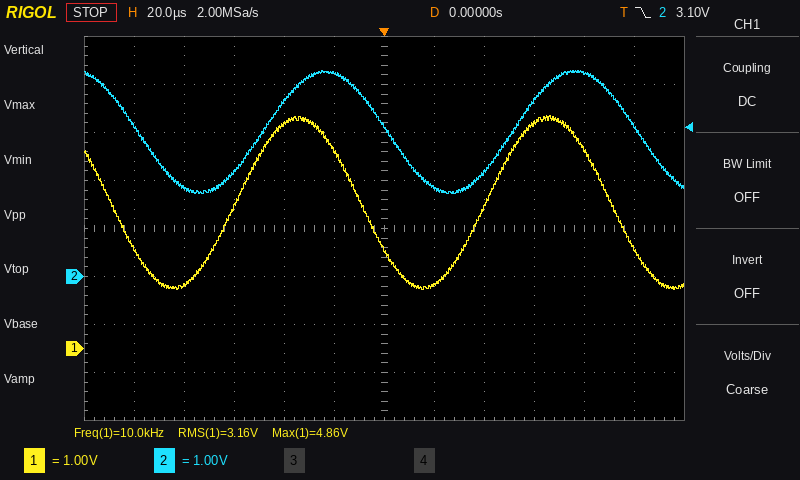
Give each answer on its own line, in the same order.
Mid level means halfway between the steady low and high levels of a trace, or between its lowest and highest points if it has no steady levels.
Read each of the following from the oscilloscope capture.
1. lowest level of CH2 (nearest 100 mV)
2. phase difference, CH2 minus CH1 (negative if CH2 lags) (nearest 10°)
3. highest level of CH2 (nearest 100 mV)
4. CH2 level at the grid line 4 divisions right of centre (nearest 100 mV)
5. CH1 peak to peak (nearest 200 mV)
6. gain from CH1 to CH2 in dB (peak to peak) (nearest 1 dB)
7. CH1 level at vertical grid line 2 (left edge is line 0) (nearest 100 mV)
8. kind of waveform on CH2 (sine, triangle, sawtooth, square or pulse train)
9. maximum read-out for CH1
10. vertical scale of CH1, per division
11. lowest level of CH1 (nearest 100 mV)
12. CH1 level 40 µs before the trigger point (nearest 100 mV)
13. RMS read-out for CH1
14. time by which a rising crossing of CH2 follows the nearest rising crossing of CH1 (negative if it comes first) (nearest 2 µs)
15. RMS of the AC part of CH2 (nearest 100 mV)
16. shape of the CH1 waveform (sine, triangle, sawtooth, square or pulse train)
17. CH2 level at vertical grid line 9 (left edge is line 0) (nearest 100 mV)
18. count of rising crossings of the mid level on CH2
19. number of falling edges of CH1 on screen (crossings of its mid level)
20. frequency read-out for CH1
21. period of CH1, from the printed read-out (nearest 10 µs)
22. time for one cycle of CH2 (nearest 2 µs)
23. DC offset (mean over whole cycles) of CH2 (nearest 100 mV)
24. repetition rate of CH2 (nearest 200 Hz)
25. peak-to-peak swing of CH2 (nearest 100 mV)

1.7 V
-40°
4.3 V
4.2 V
3.6 V
-3 dB
1.3 V
sine
4.86 V
1 V
1.2 V
4.7 V
3.16 V
+10 µs
900 mV
sine
3.7 V
2
3
10.0 kHz
100 µs
100 µs
3.0 V
10.0 kHz
2.6 V
